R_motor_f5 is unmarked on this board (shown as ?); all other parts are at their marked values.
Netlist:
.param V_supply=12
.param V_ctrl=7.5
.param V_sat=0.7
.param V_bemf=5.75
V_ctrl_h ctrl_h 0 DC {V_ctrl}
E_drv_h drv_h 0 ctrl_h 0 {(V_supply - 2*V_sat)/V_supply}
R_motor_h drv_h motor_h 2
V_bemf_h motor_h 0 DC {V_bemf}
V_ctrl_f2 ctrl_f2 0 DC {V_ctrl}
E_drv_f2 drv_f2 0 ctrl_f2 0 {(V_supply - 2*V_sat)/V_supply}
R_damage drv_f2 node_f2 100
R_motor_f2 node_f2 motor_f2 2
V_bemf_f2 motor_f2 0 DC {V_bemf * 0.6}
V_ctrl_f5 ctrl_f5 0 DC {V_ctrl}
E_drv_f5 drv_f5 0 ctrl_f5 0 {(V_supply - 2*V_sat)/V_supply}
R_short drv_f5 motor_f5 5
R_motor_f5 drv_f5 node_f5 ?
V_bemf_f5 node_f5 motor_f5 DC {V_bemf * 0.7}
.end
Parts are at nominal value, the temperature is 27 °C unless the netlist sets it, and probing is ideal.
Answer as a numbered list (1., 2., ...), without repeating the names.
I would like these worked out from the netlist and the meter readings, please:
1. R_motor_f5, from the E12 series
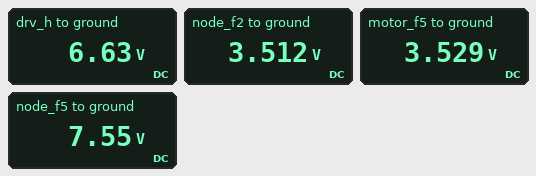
1. 1.5 Ω
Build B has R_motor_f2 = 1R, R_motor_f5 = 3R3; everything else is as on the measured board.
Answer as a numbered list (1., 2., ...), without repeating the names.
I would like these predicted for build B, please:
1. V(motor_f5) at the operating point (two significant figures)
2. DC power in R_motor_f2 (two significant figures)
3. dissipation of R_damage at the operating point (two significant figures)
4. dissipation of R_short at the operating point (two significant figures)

1. 4.2 V
2. 990 µW
3. 99 mW
4. 1.2 W
